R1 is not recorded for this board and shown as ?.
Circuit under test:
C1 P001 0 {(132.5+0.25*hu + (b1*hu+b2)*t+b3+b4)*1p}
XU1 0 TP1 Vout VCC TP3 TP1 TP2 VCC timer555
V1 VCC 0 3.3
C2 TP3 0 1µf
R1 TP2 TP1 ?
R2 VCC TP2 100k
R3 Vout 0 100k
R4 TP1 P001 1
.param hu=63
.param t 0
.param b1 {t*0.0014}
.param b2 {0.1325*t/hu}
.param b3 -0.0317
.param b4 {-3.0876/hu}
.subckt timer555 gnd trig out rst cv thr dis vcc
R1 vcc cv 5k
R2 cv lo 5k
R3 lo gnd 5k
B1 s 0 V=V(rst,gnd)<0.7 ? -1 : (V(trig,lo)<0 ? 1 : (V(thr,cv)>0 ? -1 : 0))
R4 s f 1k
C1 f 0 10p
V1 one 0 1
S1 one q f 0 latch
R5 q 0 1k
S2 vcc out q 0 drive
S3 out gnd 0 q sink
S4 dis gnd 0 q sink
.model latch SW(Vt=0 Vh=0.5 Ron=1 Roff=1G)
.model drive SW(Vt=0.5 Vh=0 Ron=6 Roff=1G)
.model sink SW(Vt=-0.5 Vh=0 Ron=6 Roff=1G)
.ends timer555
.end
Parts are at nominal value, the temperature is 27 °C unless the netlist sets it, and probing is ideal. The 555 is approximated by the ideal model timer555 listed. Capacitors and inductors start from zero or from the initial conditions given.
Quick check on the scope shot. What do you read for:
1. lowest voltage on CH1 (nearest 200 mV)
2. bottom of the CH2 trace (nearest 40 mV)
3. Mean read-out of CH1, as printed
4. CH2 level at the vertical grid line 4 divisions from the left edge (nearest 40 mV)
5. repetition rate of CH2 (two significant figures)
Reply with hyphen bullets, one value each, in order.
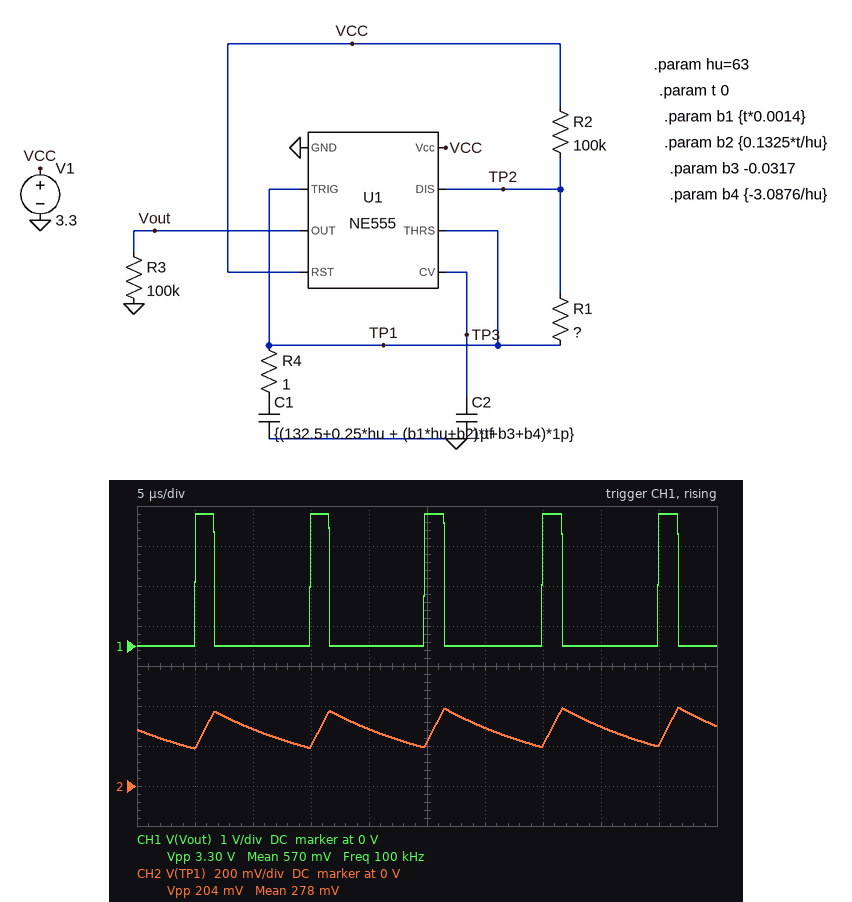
- 0 V
- 200 mV
- 570 mV
- 280 mV
- 100 kHz
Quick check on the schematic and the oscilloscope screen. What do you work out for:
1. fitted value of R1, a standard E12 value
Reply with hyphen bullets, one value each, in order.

- 82 kΩ
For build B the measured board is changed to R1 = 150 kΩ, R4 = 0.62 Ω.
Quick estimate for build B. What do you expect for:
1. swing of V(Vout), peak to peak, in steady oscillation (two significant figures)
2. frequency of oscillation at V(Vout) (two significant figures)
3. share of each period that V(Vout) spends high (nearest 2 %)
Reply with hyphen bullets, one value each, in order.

- 3.3 V
- 57 kHz
- 14 %
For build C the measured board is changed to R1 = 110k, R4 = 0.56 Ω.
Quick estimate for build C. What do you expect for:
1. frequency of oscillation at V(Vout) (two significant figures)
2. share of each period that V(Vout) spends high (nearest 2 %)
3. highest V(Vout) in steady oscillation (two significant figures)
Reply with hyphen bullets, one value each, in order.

- 76 kHz
- 16 %
- 3.3 V
